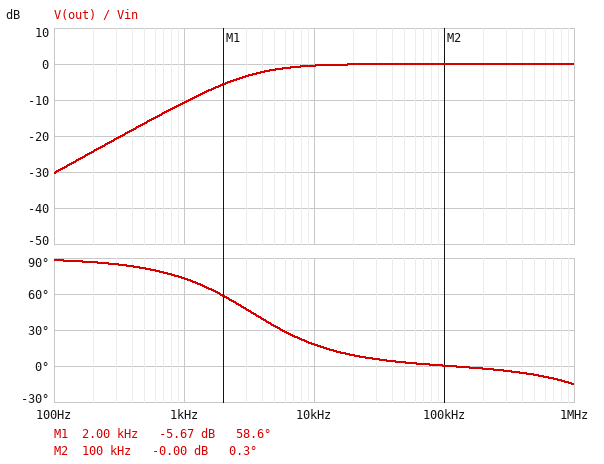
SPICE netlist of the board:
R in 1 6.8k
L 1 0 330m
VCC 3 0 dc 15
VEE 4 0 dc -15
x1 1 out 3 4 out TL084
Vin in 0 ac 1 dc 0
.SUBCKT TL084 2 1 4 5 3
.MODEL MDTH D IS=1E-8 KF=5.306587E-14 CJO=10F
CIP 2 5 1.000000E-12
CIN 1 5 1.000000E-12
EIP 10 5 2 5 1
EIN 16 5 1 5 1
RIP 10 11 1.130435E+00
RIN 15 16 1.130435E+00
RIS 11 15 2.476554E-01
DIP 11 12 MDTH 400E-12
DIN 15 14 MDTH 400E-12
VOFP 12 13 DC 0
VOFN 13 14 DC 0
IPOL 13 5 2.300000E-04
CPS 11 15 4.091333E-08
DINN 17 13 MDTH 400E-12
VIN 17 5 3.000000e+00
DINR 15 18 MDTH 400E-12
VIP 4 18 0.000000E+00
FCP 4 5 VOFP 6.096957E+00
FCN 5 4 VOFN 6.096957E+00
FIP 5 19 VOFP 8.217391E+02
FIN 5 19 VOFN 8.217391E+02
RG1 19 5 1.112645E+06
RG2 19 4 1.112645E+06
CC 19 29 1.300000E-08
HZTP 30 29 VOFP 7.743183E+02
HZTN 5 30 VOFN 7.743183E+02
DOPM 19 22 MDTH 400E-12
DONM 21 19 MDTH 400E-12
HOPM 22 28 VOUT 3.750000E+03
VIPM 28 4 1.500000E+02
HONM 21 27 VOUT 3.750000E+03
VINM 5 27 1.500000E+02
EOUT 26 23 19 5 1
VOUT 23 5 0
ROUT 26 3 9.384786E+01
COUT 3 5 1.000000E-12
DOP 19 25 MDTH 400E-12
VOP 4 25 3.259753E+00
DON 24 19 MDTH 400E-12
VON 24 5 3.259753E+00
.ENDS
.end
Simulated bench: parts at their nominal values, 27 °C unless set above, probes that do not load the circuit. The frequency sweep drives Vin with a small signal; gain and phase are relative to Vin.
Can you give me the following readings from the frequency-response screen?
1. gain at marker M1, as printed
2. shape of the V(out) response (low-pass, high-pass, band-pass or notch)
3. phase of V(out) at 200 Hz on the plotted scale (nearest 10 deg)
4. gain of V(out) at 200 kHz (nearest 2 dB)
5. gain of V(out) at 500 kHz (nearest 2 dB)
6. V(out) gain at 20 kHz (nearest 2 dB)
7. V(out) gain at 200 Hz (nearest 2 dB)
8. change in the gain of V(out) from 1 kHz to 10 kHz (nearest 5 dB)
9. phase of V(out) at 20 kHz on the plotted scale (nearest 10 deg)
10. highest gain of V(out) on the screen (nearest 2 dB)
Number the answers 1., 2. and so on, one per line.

1. -5.67 dB
2. high-pass
3. 90 deg
4. 0 dB
5. 0 dB
6. 0 dB
7. -24 dB
8. 10 dB
9. 10 deg
10. 0 dB
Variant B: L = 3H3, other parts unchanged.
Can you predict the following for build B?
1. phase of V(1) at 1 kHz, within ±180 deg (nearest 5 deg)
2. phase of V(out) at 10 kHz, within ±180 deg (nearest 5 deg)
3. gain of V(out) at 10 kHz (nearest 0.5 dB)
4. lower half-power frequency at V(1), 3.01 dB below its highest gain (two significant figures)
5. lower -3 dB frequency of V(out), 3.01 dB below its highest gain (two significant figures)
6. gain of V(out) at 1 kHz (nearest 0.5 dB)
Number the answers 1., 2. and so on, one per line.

1. 20 deg
2. 0 deg
3. 0 dB
4. 330 Hz
5. 360 Hz
6. -0.5 dB
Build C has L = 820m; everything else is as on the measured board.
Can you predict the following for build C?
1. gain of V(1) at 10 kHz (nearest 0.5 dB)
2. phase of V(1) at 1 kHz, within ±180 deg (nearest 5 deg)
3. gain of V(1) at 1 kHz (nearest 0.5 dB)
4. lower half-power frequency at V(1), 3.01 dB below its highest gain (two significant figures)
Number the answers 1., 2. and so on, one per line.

1. 0 dB
2. 55 deg
3. -4.5 dB
4. 1.3 kHz
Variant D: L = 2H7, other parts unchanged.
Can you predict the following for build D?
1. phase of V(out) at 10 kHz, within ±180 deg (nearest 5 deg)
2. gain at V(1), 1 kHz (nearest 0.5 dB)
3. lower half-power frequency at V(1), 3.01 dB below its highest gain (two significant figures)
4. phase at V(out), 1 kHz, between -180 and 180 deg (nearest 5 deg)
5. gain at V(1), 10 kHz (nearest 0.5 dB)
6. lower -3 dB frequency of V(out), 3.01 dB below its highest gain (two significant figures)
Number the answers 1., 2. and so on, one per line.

1. 0 deg
2. -0.5 dB
3. 400 Hz
4. 20 deg
5. 0 dB
6. 440 Hz
